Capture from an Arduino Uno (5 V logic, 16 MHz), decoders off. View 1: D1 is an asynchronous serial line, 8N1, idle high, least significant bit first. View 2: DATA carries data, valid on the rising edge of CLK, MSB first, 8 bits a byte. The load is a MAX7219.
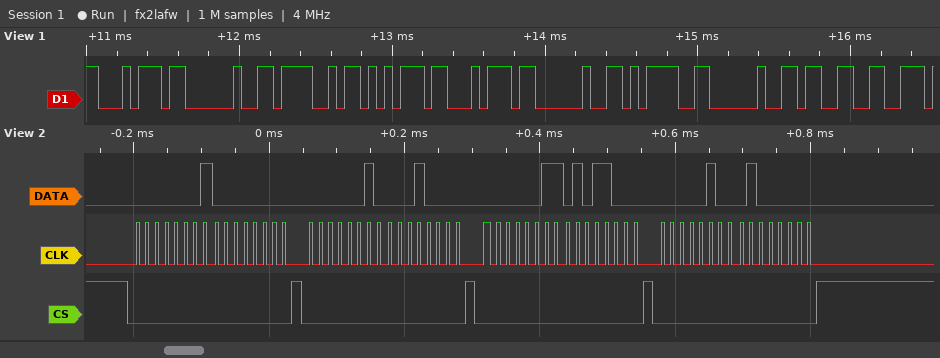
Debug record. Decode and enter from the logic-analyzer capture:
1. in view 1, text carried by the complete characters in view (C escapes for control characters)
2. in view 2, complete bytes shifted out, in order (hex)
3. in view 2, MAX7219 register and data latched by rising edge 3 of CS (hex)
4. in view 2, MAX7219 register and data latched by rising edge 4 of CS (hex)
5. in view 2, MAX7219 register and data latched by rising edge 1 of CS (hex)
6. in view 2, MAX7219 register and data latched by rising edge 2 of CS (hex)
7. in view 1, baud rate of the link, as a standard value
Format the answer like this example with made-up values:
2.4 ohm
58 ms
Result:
"t Out = 3"
01 00 02 10 03 58 04 40
register 0x3, data 0x58
register 0x4, data 0x40
register 0x1, data 0x00
register 0x2, data 0x10
19200 baud
